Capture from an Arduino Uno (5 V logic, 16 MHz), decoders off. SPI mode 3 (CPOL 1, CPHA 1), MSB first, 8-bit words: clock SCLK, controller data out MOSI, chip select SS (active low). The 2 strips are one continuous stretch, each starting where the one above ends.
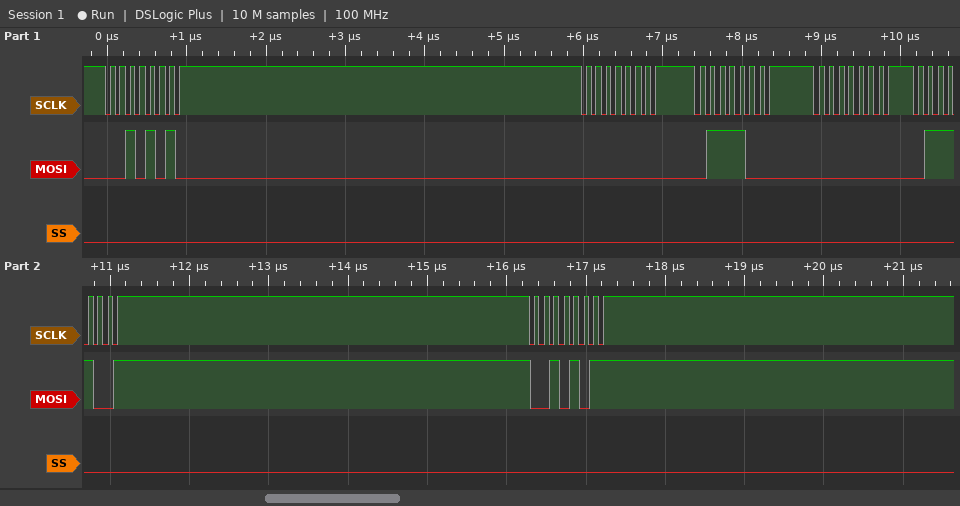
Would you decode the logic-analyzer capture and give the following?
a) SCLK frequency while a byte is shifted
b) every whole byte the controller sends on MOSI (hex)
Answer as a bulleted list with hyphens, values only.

- 8 MHz
- 2A 00 78 00 79 2B
